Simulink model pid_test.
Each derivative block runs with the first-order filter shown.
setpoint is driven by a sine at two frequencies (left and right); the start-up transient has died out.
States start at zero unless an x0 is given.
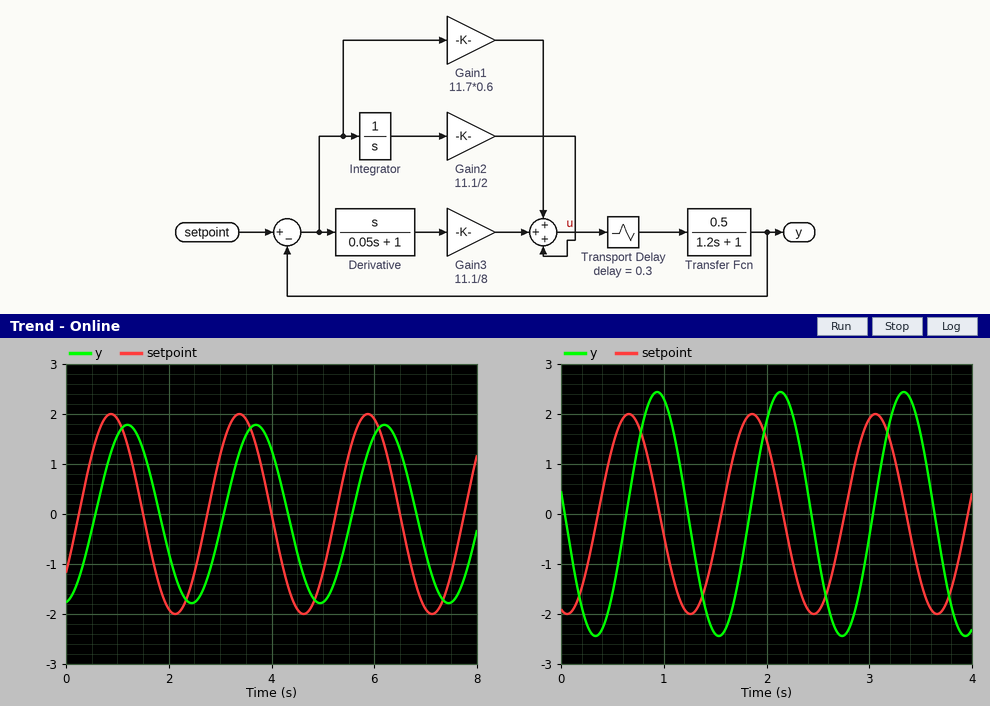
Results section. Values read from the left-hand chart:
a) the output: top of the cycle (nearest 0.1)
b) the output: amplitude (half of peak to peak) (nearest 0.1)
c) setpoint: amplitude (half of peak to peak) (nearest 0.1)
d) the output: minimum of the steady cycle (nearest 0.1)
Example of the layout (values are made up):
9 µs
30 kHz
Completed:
1.8
1.8
2.0
-1.8
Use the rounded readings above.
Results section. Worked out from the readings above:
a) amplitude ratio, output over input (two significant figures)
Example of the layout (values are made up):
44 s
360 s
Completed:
0.90
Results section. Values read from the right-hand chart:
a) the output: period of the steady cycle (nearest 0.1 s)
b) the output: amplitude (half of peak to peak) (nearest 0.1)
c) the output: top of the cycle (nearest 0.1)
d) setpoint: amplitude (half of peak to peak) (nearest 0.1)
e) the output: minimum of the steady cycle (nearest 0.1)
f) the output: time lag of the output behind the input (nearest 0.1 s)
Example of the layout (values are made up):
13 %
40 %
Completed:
1.2 s
2.4
2.4
2.0
-2.4
0.3 s
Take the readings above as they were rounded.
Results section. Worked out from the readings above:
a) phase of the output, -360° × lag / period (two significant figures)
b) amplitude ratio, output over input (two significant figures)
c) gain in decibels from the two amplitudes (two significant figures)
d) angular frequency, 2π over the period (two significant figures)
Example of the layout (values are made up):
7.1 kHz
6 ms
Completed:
-90°
1.2
1.6 dB
5.2 rad/s
